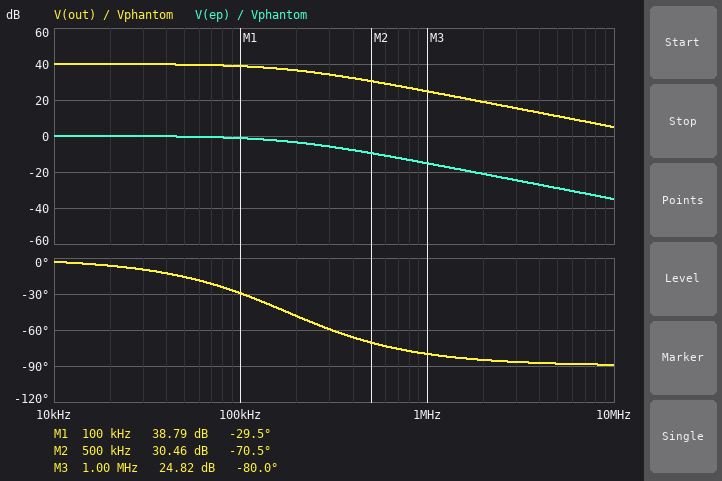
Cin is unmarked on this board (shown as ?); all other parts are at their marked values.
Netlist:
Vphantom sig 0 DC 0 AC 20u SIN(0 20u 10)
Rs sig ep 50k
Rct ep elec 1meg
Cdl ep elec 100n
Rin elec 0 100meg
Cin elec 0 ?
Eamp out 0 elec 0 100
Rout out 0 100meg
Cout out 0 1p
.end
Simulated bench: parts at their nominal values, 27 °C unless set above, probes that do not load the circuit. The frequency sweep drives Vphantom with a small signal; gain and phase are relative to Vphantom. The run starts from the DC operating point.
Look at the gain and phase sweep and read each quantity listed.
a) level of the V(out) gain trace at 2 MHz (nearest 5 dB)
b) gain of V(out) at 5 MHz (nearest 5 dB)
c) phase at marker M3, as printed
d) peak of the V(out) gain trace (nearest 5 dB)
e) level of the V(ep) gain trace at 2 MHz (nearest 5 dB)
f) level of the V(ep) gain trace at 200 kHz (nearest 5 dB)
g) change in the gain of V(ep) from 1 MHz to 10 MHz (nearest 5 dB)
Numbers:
20 dB
10 dB
-80.0 deg
40 dB
-20 dB
-5 dB
-20 dB
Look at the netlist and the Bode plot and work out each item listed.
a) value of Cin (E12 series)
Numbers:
18 pF
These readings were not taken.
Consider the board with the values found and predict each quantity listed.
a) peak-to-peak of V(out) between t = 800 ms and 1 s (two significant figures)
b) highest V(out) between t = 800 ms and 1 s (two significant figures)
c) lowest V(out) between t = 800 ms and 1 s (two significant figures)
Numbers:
4.0 mV
2.0 mV
-2.0 mV
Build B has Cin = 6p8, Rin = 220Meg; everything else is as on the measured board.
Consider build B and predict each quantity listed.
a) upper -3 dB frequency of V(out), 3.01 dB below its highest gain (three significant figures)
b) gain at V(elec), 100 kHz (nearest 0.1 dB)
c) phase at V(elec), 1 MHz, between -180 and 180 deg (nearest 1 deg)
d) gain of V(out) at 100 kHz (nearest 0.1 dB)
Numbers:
468 kHz
-0.2 dB
-65 deg
39.8 dB
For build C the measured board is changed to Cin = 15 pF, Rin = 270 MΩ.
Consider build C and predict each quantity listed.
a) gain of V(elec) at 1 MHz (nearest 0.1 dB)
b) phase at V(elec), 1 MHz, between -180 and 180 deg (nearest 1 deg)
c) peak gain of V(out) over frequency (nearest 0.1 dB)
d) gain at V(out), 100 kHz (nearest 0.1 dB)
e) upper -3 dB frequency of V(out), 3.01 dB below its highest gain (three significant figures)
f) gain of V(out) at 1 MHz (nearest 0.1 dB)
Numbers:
-13.7 dB
-78 deg
40.0 dB
39.1 dB
212 kHz
26.3 dB
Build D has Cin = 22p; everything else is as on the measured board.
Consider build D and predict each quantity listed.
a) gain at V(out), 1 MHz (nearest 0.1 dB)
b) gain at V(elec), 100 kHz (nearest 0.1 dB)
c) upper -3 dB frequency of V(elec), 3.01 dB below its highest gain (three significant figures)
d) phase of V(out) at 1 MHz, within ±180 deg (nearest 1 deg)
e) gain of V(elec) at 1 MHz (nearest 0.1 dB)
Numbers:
23.1 dB
-1.7 dB
145 kHz
-82 deg
-16.9 dB
